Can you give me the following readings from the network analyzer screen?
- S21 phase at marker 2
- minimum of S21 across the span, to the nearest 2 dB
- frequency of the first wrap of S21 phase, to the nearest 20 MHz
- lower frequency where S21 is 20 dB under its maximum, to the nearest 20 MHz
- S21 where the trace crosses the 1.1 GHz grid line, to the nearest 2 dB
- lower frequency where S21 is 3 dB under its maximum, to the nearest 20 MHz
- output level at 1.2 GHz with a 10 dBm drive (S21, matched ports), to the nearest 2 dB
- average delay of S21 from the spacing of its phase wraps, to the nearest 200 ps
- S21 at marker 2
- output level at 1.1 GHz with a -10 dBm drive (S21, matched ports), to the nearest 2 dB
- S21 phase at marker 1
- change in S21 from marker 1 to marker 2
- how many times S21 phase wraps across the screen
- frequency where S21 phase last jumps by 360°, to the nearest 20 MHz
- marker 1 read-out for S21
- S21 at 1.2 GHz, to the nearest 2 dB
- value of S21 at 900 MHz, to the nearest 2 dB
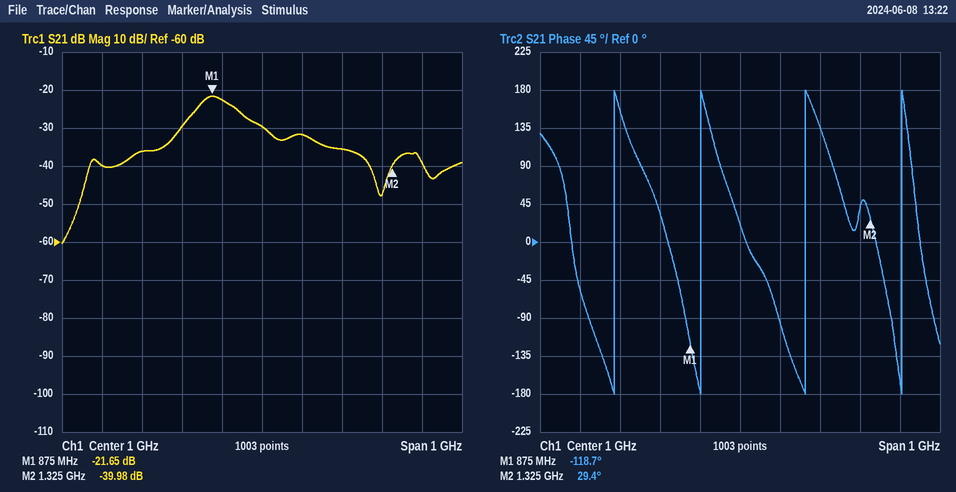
29.4°
-60 dB
680 MHz
560 MHz
-32 dB
840 MHz
-26 dBm
4.2 ns
-39.98 dB
-42 dBm
-118.7°
-18.33 dB
4
1.40 GHz
-21.65 dB
-36 dB
-22 dB
